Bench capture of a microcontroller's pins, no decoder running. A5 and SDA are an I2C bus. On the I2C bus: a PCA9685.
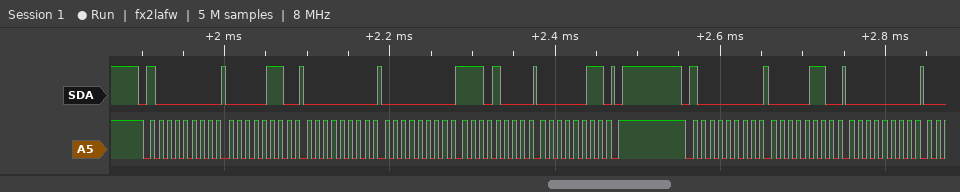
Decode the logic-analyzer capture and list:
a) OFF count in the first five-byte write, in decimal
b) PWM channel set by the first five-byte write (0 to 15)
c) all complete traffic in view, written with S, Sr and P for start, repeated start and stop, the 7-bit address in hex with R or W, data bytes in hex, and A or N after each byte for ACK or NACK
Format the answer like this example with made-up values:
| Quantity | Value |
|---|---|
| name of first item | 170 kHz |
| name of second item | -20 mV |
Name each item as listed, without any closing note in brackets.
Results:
| Quantity | Value |
|---|---|
| OFF count in the first five-byte write, in decimal | 1000 |
| PWM channel set by the first five-byte write | 0 |
| all complete traffic in view, written with S, Sr and P for start, repeated start and stop, the 7-bit address in hex with R or W, data bytes in hex, and A or N after each byte for ACK or NACK | S 40W A 06 A 00 A 00 A E8 A 03 A P S 40W A 06 A 00 A |
